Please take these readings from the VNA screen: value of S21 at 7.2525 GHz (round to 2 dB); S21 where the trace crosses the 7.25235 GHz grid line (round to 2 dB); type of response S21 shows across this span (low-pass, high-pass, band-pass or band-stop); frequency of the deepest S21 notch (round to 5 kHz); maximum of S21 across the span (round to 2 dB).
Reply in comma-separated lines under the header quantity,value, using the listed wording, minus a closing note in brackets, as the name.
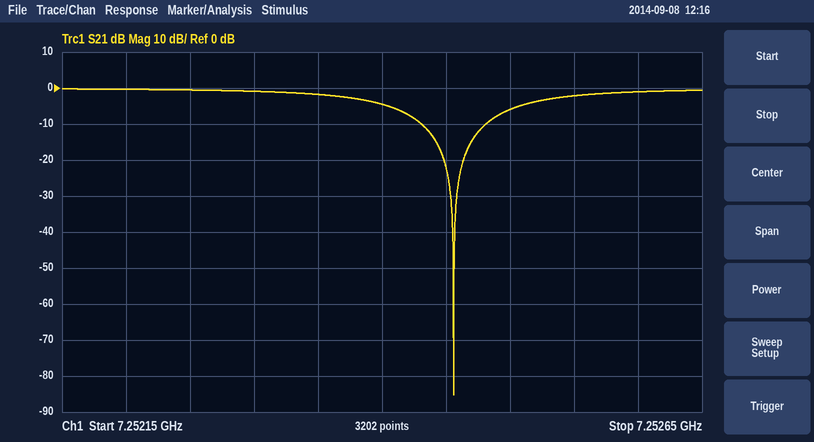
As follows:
quantity,value
value of S21 at 7.2525 GHz,-6 dB
S21 where the trace crosses the 7.25235 GHz grid line,-2 dB
type of response S21 shows across this span,band-stop
frequency of the deepest S21 notch,7.252455 GHz
maximum of S21 across the span,0 dB
